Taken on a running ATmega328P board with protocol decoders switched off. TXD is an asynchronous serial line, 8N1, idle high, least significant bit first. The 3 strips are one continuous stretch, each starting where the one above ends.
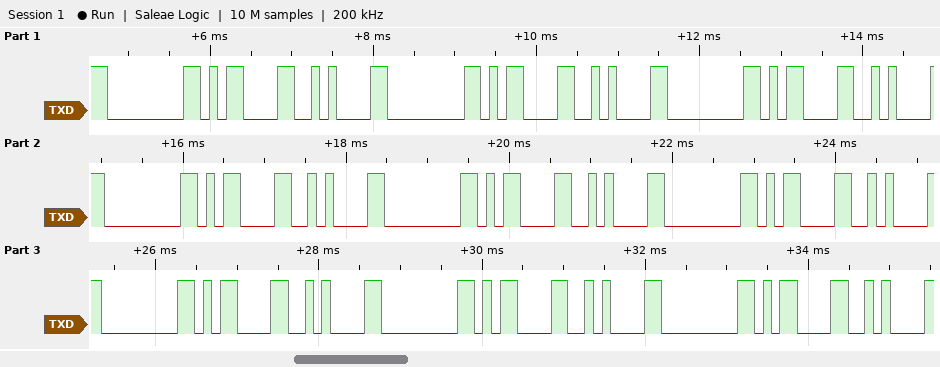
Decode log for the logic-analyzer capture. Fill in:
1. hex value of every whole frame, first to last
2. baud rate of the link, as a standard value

00 0D 0A 00 0D 0A 00 0D 0A 00 0D 0A 00 0D 0A 00 0D 0A 00 0D 0A 00 0D 0A 00 0D 0A
9600 baud
